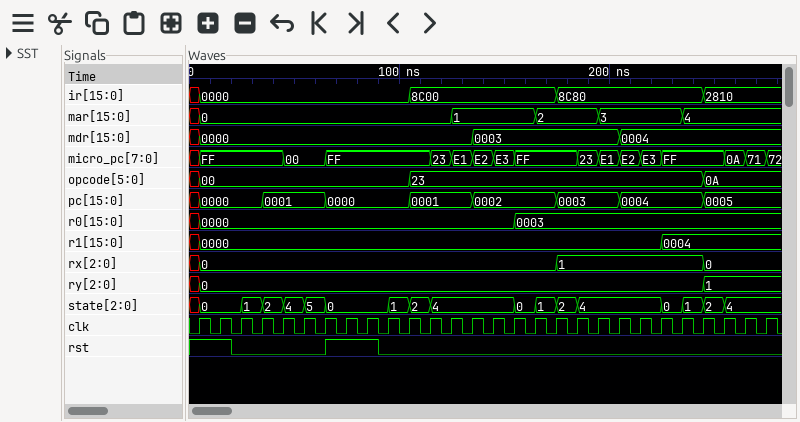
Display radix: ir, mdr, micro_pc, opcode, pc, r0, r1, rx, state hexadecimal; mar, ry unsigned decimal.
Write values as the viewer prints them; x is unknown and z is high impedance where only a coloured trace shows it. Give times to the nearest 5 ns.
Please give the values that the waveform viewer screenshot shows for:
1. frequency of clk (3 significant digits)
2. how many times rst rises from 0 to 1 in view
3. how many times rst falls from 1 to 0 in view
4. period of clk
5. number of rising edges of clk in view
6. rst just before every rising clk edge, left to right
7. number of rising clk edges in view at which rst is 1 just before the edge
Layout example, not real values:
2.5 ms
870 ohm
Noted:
100 MHz
1
2
10 ns
28
1 1 0 0 0 0 0 1 1 0 0 0 0 0 0 0 0 0 0 0 0 0 0 0 0 0 0 0
4
